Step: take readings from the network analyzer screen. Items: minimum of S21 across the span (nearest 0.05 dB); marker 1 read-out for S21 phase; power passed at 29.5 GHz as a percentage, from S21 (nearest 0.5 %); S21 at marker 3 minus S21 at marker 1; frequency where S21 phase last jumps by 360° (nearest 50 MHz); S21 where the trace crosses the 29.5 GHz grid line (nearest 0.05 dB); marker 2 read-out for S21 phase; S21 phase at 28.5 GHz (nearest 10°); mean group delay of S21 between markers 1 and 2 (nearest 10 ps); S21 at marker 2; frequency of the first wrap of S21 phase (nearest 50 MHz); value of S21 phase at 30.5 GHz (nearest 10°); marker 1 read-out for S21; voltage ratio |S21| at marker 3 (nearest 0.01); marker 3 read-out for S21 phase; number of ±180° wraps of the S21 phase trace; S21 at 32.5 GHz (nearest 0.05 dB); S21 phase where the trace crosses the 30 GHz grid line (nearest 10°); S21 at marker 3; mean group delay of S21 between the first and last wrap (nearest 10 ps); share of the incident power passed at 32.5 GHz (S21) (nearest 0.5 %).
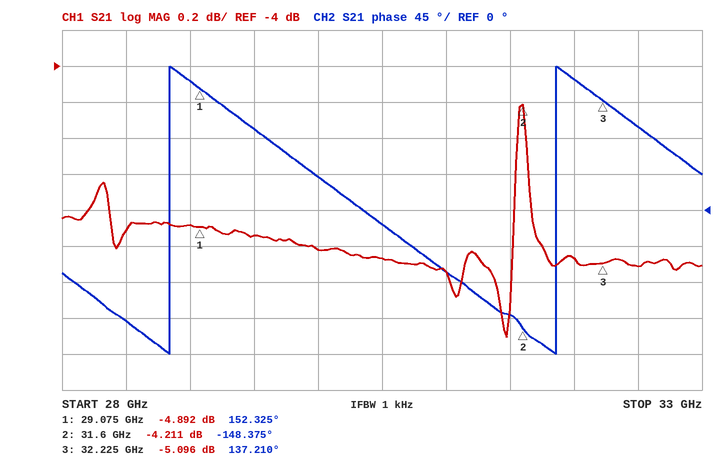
-5.50 dB
152.325°
32.0 %
-0.204 dB
31.85 GHz
-4.95 dB
-148.375°
-140°
330 ps
-4.211 dB
28.85 GHz
-20°
-4.892 dB
0.56
137.210°
2
-5.10 dB
40°
-5.096 dB
330 ps
31.0 %
